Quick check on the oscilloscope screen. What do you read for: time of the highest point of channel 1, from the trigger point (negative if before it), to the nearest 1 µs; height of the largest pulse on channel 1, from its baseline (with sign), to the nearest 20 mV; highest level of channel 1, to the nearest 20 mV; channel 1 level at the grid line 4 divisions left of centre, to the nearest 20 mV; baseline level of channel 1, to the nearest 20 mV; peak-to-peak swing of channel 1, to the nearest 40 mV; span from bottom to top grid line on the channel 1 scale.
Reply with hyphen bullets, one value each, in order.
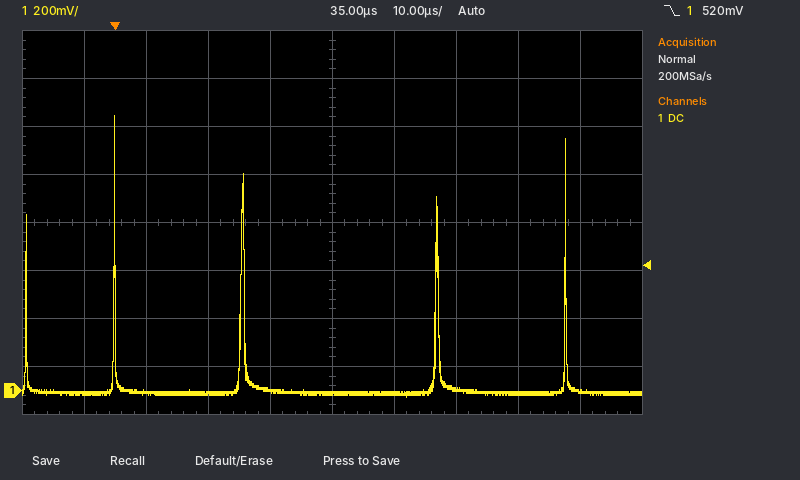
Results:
- 0 µs
- +1.16 V
- 1.14 V
- -20 mV
- -20 mV
- 1.16 V
- 1.6 V
